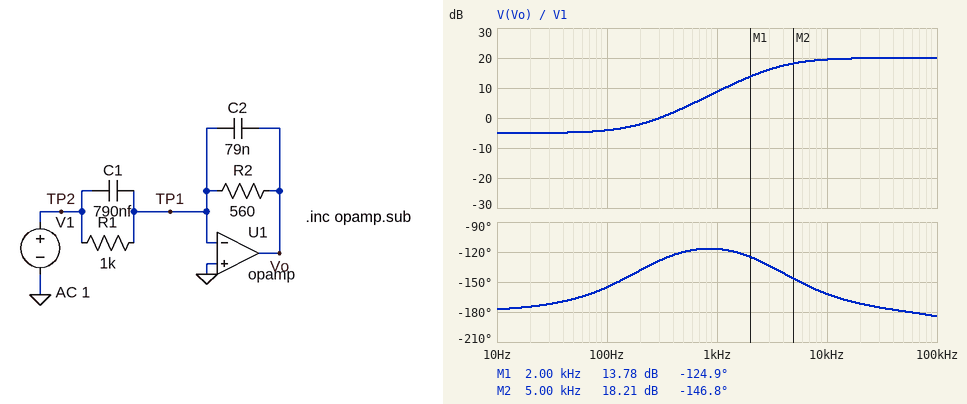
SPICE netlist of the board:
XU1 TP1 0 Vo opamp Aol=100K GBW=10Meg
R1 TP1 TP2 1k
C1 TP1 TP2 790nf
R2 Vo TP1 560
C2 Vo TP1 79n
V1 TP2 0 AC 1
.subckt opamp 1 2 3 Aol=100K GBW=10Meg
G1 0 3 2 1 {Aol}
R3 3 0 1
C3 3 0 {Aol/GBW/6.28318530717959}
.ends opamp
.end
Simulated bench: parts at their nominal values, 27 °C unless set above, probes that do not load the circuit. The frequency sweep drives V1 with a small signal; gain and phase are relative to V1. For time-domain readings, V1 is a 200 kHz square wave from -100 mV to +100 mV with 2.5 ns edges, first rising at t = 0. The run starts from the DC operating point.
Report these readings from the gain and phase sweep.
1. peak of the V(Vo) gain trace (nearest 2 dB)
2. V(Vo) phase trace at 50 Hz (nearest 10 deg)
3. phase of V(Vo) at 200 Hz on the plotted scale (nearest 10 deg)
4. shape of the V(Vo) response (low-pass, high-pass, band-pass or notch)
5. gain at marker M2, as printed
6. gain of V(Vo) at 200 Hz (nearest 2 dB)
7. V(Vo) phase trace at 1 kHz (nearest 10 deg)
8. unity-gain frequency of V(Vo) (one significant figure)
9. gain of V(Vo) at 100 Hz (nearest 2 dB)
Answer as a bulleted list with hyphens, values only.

- 20 dB
- -170 deg
- -140 deg
- high-pass
- 18.21 dB
- -2 dB
- -120 deg
- 300 Hz
- -4 dB
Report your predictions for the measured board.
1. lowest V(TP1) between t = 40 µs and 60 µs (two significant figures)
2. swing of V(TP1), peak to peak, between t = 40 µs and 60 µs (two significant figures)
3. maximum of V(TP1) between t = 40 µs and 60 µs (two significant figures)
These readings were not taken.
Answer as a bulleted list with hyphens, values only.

- -180 mV
- 360 mV
- 180 mV
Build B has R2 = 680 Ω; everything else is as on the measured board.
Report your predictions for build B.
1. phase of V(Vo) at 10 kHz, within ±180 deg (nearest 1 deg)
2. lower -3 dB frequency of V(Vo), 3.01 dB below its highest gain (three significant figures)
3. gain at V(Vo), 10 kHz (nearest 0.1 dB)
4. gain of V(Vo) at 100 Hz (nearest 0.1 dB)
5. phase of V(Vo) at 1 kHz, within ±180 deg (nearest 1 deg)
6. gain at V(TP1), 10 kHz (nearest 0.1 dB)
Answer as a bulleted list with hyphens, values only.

- -165 deg
- 2.94 kHz
- 19.7 dB
- -2.4 dB
- -120 deg
- -40.3 dB
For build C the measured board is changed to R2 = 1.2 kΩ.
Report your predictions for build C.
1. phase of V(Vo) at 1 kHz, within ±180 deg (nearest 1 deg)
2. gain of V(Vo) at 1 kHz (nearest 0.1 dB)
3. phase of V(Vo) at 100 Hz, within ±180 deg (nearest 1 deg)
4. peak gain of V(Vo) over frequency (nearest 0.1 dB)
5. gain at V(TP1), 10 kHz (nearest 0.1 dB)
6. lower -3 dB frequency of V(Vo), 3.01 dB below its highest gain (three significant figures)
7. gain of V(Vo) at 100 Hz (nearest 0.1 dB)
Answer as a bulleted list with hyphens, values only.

- -132 deg
- 14.4 dB
- -157 deg
- 20.0 dB
- -40.1 dB
- 1.65 kHz
- 2.5 dB
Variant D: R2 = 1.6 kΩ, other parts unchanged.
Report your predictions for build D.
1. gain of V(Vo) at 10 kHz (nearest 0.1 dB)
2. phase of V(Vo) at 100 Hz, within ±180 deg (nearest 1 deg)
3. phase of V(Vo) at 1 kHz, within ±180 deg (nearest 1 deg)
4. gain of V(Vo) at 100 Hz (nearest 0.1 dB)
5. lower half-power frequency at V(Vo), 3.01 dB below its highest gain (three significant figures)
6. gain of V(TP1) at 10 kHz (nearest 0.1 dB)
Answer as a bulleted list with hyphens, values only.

- 19.9 dB
- -158 deg
- -140 deg
- 5.0 dB
- 1.22 kHz
- -40.1 dB
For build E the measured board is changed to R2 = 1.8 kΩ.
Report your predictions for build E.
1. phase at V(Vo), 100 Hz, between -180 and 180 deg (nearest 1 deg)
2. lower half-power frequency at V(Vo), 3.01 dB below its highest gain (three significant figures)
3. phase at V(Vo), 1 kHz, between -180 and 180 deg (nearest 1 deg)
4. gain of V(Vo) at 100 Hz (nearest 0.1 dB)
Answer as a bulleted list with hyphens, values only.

- -159 deg
- 1.08 kHz
- -143 deg
- 6.0 dB
